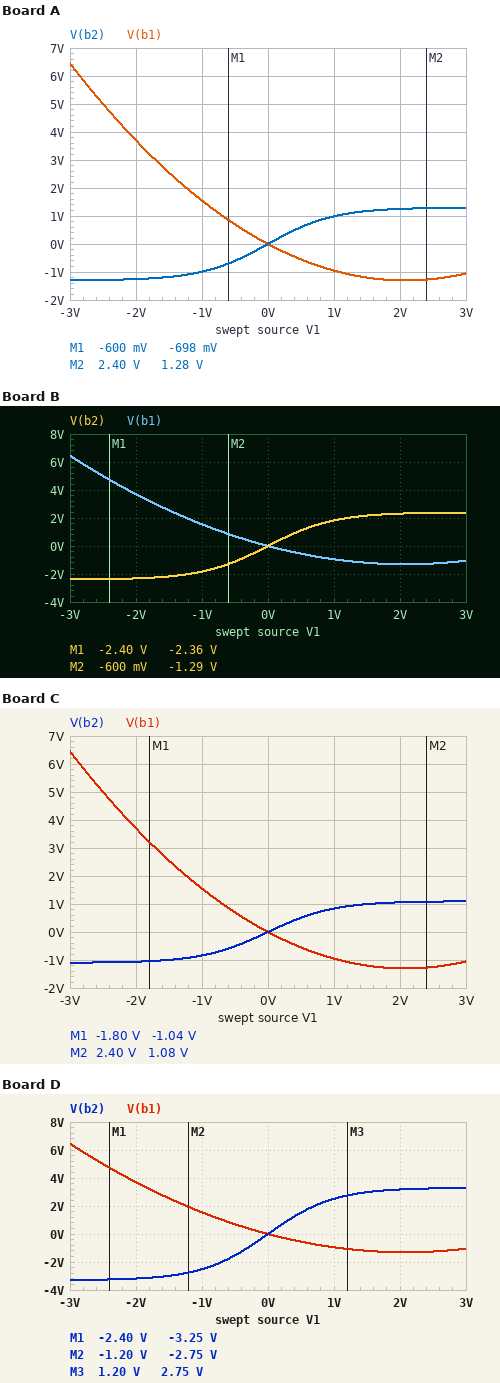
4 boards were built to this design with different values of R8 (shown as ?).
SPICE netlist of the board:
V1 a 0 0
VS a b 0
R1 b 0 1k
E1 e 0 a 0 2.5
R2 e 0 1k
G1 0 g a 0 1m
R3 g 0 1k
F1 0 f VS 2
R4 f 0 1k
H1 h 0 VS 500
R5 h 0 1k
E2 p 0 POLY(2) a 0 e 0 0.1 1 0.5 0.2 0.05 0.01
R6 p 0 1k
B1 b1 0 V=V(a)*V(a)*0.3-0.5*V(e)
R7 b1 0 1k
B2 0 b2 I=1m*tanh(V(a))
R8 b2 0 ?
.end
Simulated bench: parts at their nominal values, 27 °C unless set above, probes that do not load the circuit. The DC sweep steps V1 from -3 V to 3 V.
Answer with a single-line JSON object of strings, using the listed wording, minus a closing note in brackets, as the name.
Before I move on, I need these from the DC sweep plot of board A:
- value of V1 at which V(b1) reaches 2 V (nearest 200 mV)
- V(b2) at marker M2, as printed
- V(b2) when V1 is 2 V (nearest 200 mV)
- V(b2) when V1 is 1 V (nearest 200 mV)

{"value of V1 at which V(b1) reaches 2 V": "-1.2 V", "V(b2) at marker M2, as printed": "1.28 V", "V(b2) when V1 is 2 V": "1.2 V", "V(b2) when V1 is 1 V": "1.0 V"}
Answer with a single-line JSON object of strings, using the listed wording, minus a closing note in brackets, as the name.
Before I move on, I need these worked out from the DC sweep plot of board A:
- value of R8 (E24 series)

{"value of R8": "1.3 kΩ"}
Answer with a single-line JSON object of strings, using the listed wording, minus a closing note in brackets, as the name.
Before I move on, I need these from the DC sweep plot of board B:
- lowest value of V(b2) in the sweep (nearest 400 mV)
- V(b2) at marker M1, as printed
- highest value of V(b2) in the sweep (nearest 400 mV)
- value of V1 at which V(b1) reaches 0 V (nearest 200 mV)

{"lowest value of V(b2) in the sweep": "-2.4 V", "V(b2) at marker M1, as printed": "-2.36 V", "highest value of V(b2) in the sweep": "2.4 V", "value of V1 at which V(b1) reaches 0 V": "0 V"}
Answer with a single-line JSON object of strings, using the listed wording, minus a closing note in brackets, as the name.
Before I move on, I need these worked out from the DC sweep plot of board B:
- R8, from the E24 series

{"R8, from the E24 series": "2.4 kΩ"}
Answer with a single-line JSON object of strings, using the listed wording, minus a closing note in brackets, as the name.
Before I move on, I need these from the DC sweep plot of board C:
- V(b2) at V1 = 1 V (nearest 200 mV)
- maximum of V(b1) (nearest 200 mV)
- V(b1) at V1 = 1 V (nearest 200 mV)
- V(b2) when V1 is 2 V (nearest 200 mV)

{"V(b2) at V1 = 1 V": "800 mV", "maximum of V(b1)": "6.4 V", "V(b1) at V1 = 1 V": "-1.0 V", "V(b2) when V1 is 2 V": "1.0 V"}
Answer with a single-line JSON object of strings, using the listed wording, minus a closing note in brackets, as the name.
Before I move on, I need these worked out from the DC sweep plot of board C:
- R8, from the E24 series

{"R8, from the E24 series": "1.1 kΩ"}
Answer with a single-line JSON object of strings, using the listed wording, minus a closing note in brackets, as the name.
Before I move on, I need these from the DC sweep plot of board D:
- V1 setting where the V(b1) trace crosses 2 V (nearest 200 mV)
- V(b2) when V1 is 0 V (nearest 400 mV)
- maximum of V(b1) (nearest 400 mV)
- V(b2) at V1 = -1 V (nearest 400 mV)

{"V1 setting where the V(b1) trace crosses 2 V": "-1.2 V", "V(b2) when V1 is 0 V": "0 V", "maximum of V(b1)": "6.4 V", "V(b2) at V1 = -1 V": "-2.4 V"}
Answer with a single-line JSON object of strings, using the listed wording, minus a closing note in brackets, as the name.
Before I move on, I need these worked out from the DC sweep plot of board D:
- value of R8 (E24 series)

{"value of R8": "3.3 kΩ"}
